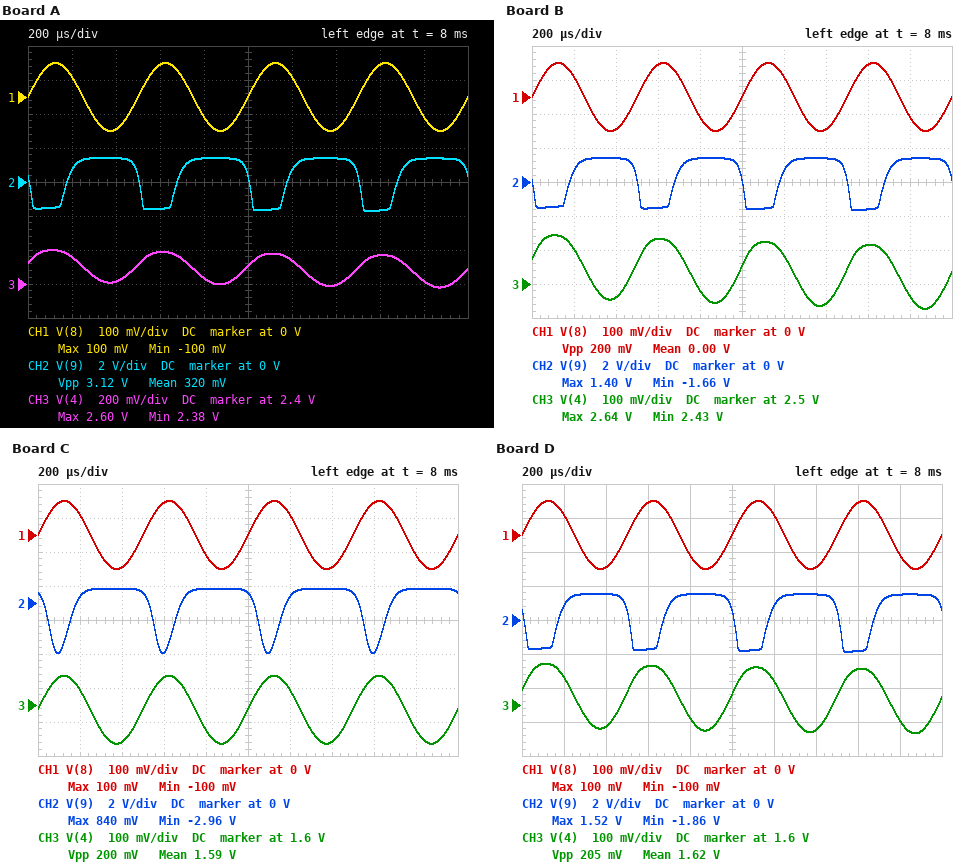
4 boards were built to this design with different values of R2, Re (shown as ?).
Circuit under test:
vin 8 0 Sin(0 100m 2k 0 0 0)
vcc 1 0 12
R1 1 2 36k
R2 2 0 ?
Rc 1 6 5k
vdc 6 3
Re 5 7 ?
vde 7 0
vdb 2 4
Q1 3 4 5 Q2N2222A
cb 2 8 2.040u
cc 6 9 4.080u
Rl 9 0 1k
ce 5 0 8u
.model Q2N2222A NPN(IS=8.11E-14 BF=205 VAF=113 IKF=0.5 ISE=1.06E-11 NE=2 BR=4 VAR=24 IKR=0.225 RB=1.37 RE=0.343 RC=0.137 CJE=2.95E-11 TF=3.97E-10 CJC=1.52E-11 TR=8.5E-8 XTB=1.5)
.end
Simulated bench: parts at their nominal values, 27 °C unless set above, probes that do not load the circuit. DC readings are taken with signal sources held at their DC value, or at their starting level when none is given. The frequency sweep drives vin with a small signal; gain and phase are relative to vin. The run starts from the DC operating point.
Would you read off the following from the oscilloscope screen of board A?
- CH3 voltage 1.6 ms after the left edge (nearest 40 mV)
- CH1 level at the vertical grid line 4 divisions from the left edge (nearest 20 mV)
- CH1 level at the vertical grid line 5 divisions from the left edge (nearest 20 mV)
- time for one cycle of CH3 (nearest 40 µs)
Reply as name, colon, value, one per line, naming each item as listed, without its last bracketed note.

CH3 voltage 1.6 ms after the left edge: 2.56 V
CH1 level at the vertical grid line 4 divisions from the left edge: -60 mV
CH1 level at the vertical grid line 5 divisions from the left edge: 0 V
time for one cycle of CH3: 520 µs
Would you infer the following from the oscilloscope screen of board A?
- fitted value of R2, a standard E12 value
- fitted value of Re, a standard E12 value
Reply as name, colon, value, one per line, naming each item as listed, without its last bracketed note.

fitted value of R2, a standard E12 value: 15 kΩ
fitted value of Re, a standard E12 value: 1.2 kΩ
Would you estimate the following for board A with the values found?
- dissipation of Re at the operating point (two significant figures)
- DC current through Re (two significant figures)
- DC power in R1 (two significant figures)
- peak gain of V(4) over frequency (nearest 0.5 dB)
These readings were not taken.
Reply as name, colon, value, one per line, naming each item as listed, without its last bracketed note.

dissipation of Re at the operating point: 4.6 mW
DC current through Re: 2.0 mA
DC power in R1: 2.3 mW
peak gain of V(4) over frequency: 0 dB
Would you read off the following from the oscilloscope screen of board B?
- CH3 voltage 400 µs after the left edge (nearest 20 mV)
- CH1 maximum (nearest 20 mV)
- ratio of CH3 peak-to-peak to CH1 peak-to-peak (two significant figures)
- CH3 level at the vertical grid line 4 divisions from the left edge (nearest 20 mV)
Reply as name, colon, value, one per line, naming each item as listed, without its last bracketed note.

CH3 voltage 400 µs after the left edge: 2.46 V
CH1 maximum: 100 mV
ratio of CH3 peak-to-peak to CH1 peak-to-peak: 1.1
CH3 level at the vertical grid line 4 divisions from the left edge: 2.48 V
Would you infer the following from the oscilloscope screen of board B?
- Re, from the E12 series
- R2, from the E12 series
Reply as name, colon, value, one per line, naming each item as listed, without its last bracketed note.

Re, from the E12 series: 1.2 kΩ
R2, from the E12 series: 18 kΩ
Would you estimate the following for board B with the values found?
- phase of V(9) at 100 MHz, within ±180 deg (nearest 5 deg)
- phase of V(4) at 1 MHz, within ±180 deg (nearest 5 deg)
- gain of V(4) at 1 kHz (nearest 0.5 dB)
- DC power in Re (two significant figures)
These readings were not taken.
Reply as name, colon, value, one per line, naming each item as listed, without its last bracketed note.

phase of V(9) at 100 MHz, within ±180 deg: 5 deg
phase of V(4) at 1 MHz, within ±180 deg: 0 deg
gain of V(4) at 1 kHz: -5.0 dB
DC power in Re: 4.8 mW
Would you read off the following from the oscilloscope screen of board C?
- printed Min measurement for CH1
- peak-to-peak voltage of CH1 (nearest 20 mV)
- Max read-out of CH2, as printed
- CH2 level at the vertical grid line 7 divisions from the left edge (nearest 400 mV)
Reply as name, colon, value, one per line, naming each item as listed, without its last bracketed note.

printed Min measurement for CH1: -100 mV
peak-to-peak voltage of CH1: 200 mV
Max read-out of CH2, as printed: 840 mV
CH2 level at the vertical grid line 7 divisions from the left edge: 800 mV
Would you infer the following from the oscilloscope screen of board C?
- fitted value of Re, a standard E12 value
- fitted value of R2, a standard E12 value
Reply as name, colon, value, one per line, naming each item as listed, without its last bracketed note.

fitted value of Re, a standard E12 value: 1 kΩ
fitted value of R2, a standard E12 value: 5.6 kΩ
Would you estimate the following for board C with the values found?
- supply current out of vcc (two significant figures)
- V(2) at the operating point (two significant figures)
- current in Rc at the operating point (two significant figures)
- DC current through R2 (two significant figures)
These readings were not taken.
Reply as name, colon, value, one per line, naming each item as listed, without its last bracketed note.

supply current out of vcc: 1.3 mA
V(2) at the operating point: 1.6 V
current in Rc at the operating point: 980 µA
DC current through R2: 280 µA
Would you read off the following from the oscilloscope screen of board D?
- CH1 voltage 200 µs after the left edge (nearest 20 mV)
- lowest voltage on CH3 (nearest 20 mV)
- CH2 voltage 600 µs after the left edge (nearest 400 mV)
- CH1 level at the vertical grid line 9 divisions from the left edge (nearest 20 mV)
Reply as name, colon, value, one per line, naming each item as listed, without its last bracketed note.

CH1 voltage 200 µs after the left edge: 60 mV
lowest voltage on CH3: 1.52 V
CH2 voltage 600 µs after the left edge: -1.6 V
CH1 level at the vertical grid line 9 divisions from the left edge: -60 mV
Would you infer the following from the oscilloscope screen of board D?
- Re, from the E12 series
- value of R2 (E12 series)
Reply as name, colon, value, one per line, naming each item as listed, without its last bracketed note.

Re, from the E12 series: 680 Ω
value of R2: 8.2 kΩ
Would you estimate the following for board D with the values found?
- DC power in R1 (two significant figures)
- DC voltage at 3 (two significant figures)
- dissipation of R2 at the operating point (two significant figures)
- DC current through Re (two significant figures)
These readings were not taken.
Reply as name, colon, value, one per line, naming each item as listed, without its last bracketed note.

DC power in R1: 2.7 mW
DC voltage at 3: 1.5 V
dissipation of R2 at the operating point: 520 µW
DC current through Re: 2.1 mA
